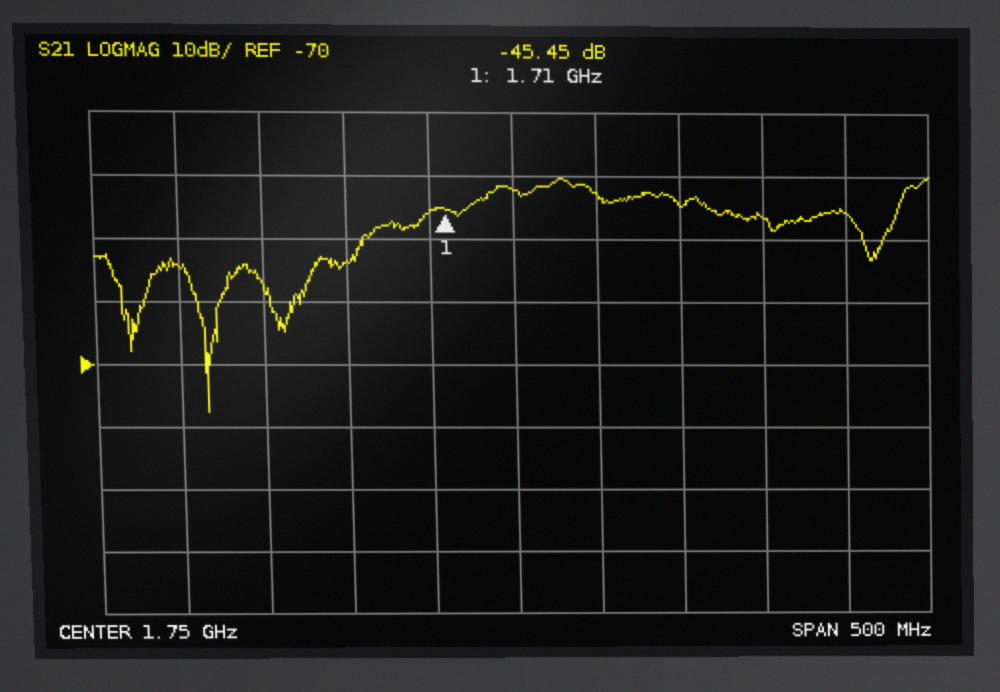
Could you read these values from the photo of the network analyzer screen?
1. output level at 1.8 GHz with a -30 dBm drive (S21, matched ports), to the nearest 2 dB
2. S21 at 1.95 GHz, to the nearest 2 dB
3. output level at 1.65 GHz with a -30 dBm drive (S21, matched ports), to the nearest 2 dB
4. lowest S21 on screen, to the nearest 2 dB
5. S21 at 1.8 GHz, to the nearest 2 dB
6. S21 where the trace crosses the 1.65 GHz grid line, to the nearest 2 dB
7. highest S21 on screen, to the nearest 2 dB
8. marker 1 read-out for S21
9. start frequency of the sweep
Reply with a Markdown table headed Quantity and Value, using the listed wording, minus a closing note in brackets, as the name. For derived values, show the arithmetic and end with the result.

| Quantity | Value |
|---|---|
| output level at 1.8 GHz with a -30 dBm drive (S21, matched ports), to the nearest 2 dB | -30 dBm + (-42 dB) = -72 dBm |
| S21 at 1.95 GHz, to the nearest 2 dB | -46 dB |
| output level at 1.65 GHz with a -30 dBm drive (S21, matched ports), to the nearest 2 dB | -30 dBm + (-54 dB) = -84 dBm |
| lowest S21 on screen, to the nearest 2 dB | -78 dB |
| S21 at 1.8 GHz, to the nearest 2 dB | -42 dB |
| S21 where the trace crosses the 1.65 GHz grid line, to the nearest 2 dB | -54 dB |
| highest S21 on screen, to the nearest 2 dB | -40 dB |
| marker 1 read-out for S21 | -45.45 dB |
| start frequency of the sweep | 1.5 GHz |
